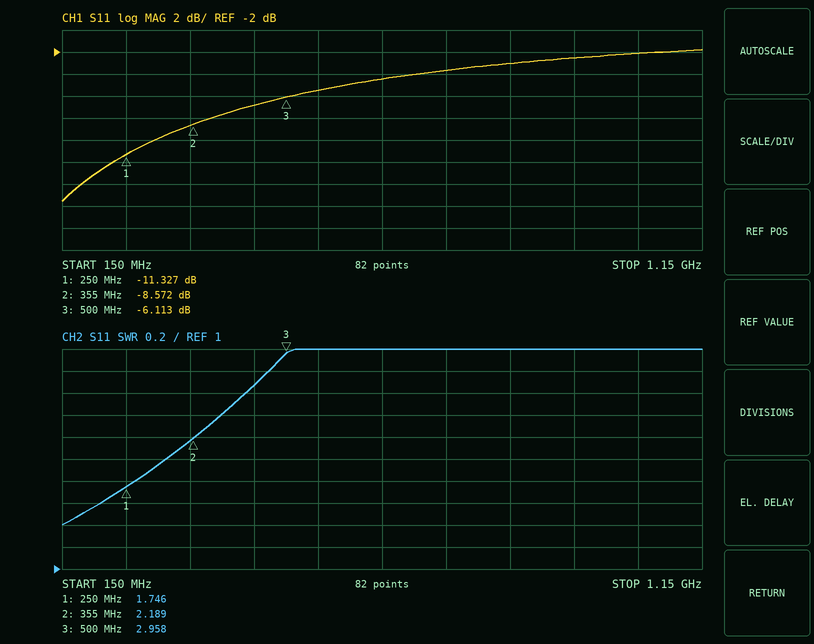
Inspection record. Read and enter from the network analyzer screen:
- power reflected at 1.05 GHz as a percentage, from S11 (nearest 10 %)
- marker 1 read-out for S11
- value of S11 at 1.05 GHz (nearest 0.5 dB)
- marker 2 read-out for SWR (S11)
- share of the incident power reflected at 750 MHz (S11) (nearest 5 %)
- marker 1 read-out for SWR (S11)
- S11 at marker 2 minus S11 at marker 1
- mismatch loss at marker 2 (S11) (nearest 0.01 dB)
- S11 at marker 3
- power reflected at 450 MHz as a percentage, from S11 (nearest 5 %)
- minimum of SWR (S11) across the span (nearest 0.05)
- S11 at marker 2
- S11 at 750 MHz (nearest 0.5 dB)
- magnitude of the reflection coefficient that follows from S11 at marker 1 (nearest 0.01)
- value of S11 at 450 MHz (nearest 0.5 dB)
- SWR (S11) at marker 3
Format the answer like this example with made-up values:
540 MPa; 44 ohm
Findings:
60 %; -11.327 dB; -2.0 dB; 2.189; 45 %; 1.746; 2.755 dB; 0.65 dB; -6.113 dB; 20 %; 1.40; -8.572 dB; -3.5 dB; 0.27; -7.0 dB; 2.958
